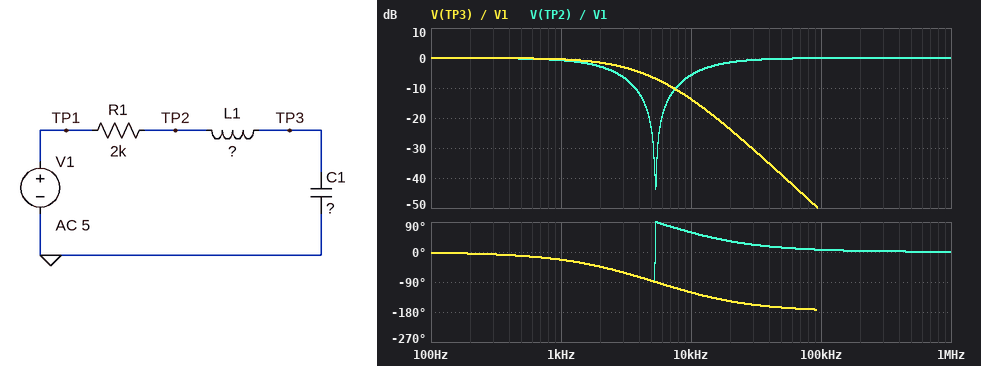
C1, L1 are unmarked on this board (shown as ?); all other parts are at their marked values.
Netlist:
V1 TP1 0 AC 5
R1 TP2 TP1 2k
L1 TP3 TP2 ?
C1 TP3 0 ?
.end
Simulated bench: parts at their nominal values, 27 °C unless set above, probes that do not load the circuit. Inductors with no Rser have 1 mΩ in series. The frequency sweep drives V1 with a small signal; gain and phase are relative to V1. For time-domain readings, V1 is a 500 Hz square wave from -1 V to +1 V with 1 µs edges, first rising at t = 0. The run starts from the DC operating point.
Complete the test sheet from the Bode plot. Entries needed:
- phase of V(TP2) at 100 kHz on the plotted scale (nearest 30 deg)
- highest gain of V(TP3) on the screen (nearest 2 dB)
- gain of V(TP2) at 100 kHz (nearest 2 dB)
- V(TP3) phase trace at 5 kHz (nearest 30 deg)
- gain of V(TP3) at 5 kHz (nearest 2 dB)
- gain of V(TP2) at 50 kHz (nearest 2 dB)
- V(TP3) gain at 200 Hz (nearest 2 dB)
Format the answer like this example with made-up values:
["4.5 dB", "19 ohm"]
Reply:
["0 deg", "0 dB", "0 dB", "-90 deg", "-6 dB", "0 dB", "0 dB"]
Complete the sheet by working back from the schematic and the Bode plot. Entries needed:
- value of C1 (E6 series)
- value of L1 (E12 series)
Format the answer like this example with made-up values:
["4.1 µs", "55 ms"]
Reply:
["33 nF", "27 mH"]
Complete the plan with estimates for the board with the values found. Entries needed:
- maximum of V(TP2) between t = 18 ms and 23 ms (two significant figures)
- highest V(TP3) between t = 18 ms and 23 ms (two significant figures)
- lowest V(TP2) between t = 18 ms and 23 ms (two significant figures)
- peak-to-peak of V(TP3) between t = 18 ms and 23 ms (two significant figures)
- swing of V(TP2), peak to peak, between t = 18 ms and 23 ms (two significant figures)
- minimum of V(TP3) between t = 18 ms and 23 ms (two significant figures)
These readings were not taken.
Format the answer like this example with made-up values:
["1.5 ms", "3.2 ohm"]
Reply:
["1.0 V", "1.0 V", "-1.0 V", "2.0 V", "2.0 V", "-1.0 V"]
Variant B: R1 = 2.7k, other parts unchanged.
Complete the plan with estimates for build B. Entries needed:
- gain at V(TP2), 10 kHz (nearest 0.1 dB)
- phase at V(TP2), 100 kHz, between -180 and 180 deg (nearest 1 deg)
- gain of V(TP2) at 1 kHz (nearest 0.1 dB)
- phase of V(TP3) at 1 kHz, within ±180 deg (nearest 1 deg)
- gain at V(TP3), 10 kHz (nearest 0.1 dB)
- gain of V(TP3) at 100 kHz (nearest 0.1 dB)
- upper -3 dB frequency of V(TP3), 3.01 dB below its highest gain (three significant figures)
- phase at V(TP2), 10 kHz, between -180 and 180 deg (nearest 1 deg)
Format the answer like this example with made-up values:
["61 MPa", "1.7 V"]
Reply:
["-7.7 dB", "9 deg", "-1.3 dB", "-30 deg", "-15.8 dB", "-51.0 dB", "2.01 kHz", "66 deg"]
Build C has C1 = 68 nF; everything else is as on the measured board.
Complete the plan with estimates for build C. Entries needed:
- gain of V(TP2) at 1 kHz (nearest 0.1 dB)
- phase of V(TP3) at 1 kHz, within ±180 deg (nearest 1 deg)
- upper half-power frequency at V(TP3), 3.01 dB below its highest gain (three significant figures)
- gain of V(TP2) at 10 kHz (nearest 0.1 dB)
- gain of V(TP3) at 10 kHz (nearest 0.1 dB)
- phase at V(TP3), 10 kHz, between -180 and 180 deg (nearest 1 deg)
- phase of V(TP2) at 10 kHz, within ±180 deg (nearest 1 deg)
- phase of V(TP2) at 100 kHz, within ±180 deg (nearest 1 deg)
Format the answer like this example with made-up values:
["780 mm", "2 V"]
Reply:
["-2.7 dB", "-43 deg", "1.30 kHz", "-4.6 dB", "-20.5 dB", "-126 deg", "54 deg", "7 deg"]
